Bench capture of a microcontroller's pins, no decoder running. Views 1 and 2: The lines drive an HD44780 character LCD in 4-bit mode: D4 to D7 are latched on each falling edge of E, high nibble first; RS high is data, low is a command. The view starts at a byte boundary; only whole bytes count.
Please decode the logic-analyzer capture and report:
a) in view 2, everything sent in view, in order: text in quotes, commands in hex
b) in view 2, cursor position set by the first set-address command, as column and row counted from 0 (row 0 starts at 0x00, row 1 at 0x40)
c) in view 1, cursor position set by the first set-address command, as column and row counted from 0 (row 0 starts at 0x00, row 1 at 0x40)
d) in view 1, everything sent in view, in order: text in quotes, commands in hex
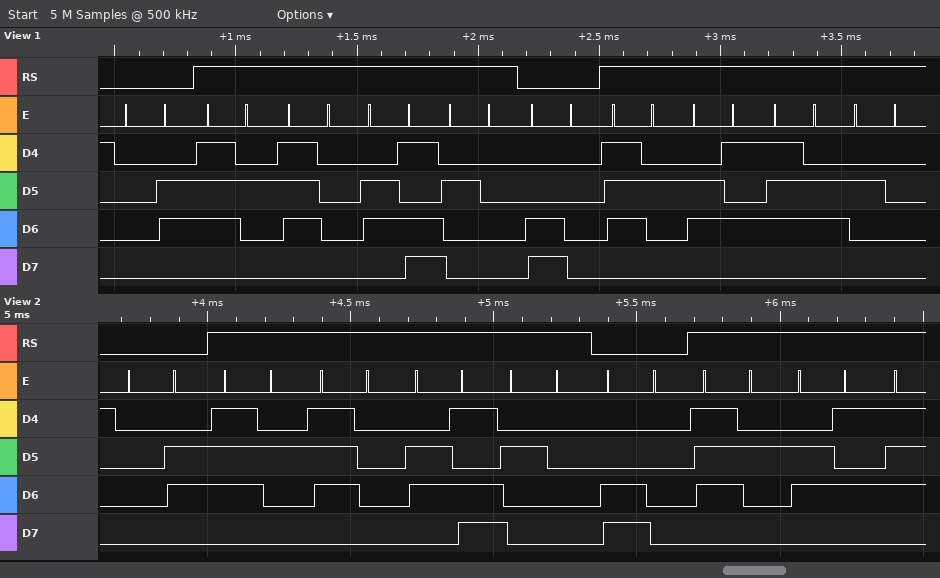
0x06 "rpm " 0xC0 "re"
column 0, row 1
column 0, row 1
0x06 "rpm " 0xC0 "rev "
